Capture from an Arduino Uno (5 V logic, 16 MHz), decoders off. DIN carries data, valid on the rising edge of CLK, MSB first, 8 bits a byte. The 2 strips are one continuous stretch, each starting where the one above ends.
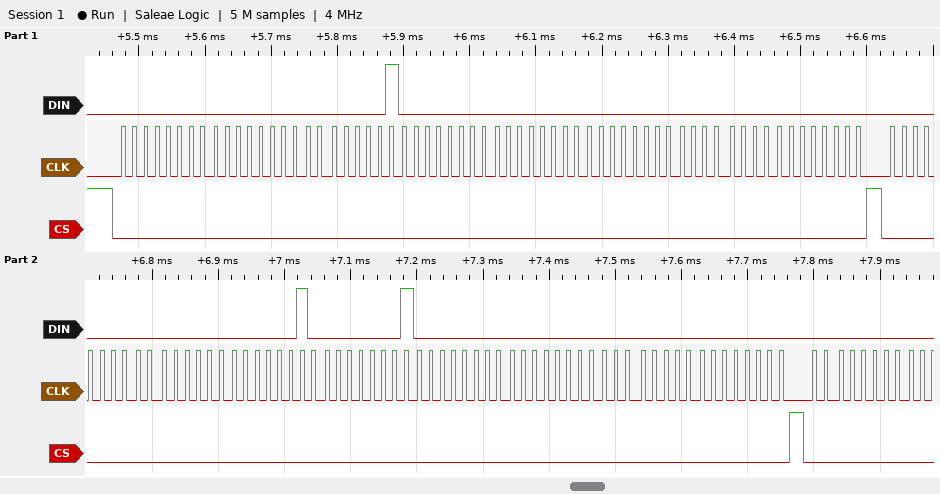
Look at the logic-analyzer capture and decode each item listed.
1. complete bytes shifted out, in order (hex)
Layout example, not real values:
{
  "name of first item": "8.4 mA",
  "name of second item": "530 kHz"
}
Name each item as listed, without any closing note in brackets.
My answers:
{
  "complete bytes shifted out, in order": "00 00 01 00 00 00 00 00 00 00 02 01 00 00 00 00 00"
}
